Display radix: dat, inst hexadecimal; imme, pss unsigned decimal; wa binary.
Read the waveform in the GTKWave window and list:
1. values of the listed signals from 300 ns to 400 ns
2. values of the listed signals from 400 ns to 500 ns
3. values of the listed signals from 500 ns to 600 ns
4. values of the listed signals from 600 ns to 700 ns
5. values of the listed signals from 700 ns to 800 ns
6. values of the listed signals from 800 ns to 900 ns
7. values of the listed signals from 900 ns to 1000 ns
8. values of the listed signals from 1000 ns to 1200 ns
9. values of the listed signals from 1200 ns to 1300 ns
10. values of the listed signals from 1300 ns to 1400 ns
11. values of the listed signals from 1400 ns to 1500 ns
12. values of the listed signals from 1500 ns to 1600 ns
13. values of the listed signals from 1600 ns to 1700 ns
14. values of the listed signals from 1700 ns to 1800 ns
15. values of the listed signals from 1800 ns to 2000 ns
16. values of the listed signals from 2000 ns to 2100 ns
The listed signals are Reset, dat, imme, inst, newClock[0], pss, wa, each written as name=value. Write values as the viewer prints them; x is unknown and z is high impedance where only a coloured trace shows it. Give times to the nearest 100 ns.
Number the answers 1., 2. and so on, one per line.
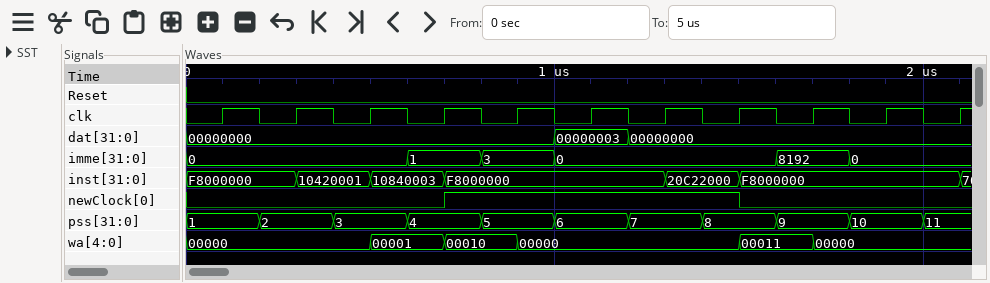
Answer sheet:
1. Reset=0, dat=00000000, imme=0, inst=10420001, newClock[0]=0, pss=2, wa=00000
2. Reset=0, dat=00000000, imme=0, inst=10420001, newClock[0]=0, pss=3, wa=00000
3. Reset=0, dat=00000000, imme=0, inst=10840003, newClock[0]=0, pss=3, wa=00001
4. Reset=0, dat=00000000, imme=1, inst=10840003, newClock[0]=0, pss=4, wa=00001
5. Reset=0, dat=00000000, imme=1, inst=F8000000, newClock[0]=1, pss=4, wa=00010
6. Reset=0, dat=00000000, imme=3, inst=F8000000, newClock[0]=1, pss=5, wa=00010
7. Reset=0, dat=00000000, imme=3, inst=F8000000, newClock[0]=1, pss=5, wa=00000
8. Reset=0, dat=00000003, imme=0, inst=F8000000, newClock[0]=1, pss=6, wa=00000
9. Reset=0, dat=00000000, imme=0, inst=F8000000, newClock[0]=1, pss=7, wa=00000
10. Reset=0, dat=00000000, imme=0, inst=20C22000, newClock[0]=1, pss=7, wa=00000
11. Reset=0, dat=00000000, imme=0, inst=20C22000, newClock[0]=1, pss=8, wa=00000
12. Reset=0, dat=00000000, imme=0, inst=F8000000, newClock[0]=0, pss=8, wa=00011
13. Reset=0, dat=00000000, imme=8192, inst=F8000000, newClock[0]=0, pss=9, wa=00011
14. Reset=0, dat=00000000, imme=8192, inst=F8000000, newClock[0]=0, pss=9, wa=00000
15. Reset=0, dat=00000000, imme=0, inst=F8000000, newClock[0]=0, pss=10, wa=00000
16. Reset=0, dat=00000000, imme=0, inst=F8000000, newClock[0]=0, pss=11, wa=00000
